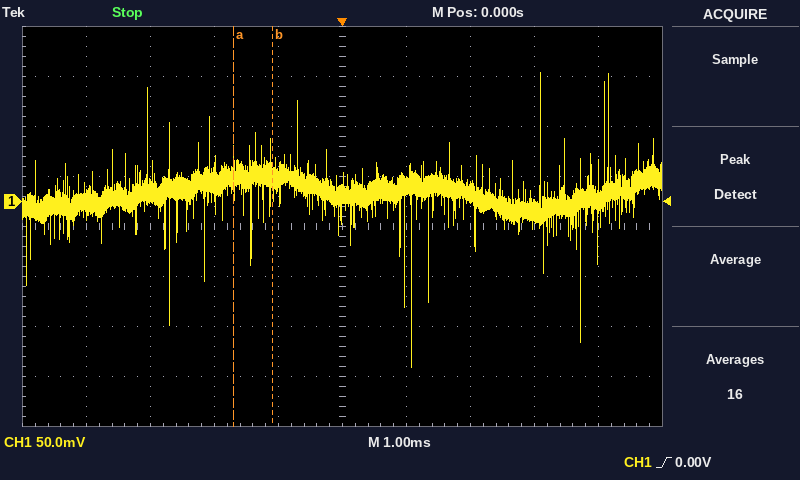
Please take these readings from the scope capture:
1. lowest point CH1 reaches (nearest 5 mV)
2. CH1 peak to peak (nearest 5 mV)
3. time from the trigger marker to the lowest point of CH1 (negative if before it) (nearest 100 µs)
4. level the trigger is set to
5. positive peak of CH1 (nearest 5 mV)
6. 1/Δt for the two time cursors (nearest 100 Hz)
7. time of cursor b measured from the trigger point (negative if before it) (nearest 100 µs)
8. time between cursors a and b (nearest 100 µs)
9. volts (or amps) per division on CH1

-165 mV
295 mV
+1.1 ms
0.00 V
130 mV
1.7 kHz
-1.1 ms
600 µs
50 mV
